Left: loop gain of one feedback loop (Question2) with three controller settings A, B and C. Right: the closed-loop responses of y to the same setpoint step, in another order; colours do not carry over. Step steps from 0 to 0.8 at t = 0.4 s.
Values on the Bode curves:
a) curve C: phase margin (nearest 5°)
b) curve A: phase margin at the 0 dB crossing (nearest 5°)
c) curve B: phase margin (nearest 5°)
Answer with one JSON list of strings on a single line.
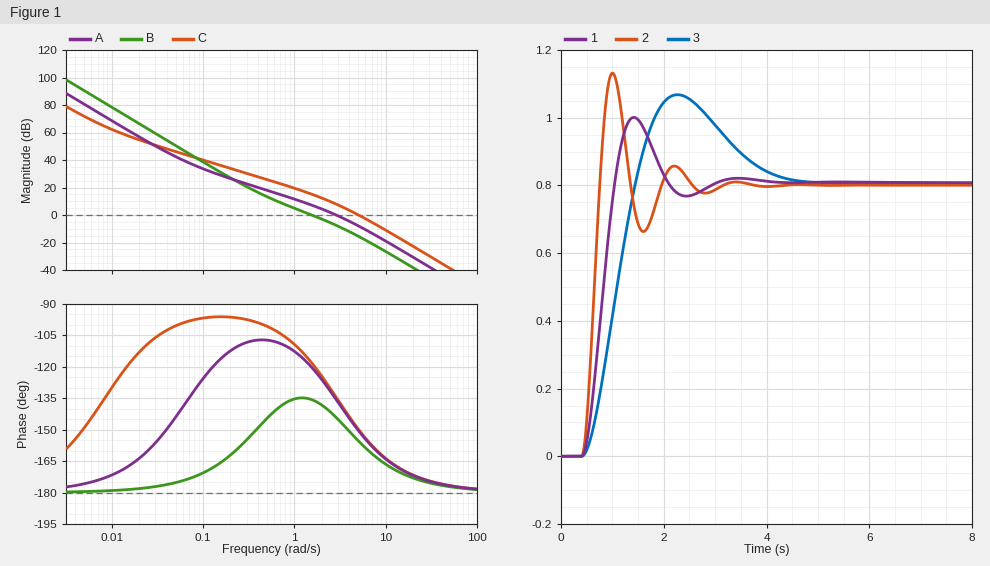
["30°", "45°", "45°"]
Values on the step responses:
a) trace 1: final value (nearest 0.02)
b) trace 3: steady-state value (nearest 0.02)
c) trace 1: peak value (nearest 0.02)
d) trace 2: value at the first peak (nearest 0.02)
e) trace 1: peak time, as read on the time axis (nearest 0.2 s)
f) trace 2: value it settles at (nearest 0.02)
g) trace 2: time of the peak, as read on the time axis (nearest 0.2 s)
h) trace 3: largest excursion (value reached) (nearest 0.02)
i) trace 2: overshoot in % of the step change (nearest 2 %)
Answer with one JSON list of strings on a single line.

["0.80", "0.80", "1.00", "1.14", "1.4 s", "0.80", "1.0 s", "1.06", "42 %"]
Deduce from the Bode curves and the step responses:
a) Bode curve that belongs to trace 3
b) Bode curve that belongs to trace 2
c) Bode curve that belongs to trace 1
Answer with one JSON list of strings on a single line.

["B", "C", "A"]
